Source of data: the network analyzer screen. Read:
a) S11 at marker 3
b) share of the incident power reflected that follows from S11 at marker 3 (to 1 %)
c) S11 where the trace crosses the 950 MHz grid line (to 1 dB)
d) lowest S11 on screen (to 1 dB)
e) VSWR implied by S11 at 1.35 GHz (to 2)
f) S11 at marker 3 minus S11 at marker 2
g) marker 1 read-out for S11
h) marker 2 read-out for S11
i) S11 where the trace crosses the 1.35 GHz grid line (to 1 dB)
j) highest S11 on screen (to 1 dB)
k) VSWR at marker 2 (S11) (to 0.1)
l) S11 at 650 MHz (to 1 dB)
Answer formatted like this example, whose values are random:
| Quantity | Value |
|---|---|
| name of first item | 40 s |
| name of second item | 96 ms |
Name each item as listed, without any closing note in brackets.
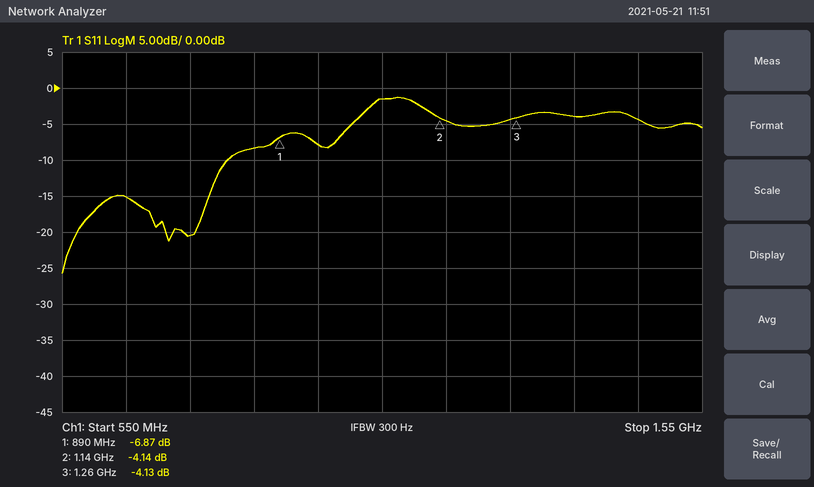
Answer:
| Quantity | Value |
|---|---|
| S11 at marker 3 | -4.13 dB |
| share of the incident power reflected that follows from S11 at marker 3 | 39 % |
| S11 where the trace crosses the 950 MHz grid line | -8 dB |
| lowest S11 on screen | -26 dB |
| VSWR implied by S11 at 1.35 GHz | 4 |
| S11 at marker 3 minus S11 at marker 2 | 0.01 dB |
| marker 1 read-out for S11 | -6.87 dB |
| marker 2 read-out for S11 | -4.14 dB |
| S11 where the trace crosses the 1.35 GHz grid line | -4 dB |
| highest S11 on screen | -1 dB |
| VSWR at marker 2 (S11) | 4.3 |
| S11 at 650 MHz | -15 dB |
